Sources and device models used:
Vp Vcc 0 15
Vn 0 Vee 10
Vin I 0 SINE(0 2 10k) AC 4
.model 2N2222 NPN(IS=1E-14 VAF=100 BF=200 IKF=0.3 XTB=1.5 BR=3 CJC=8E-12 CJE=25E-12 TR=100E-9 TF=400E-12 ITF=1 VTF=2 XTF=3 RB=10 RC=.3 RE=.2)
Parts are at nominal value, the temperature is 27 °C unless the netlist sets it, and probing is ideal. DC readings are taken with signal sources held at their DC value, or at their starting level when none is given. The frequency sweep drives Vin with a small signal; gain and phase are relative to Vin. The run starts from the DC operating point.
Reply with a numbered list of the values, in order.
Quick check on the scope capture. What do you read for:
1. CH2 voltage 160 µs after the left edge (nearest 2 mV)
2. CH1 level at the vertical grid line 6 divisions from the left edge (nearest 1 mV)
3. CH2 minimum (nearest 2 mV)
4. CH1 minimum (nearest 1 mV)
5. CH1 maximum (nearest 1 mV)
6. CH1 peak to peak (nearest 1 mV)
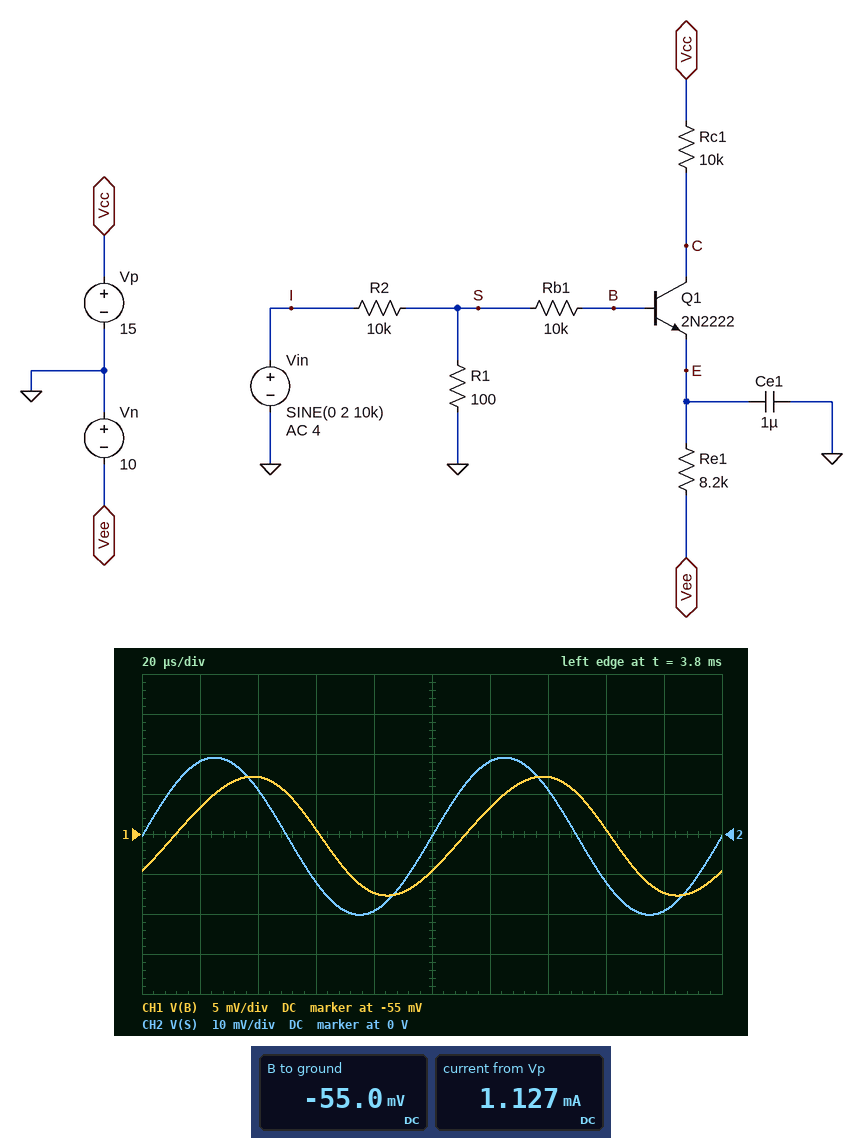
1. -12 mV
2. -52 mV
3. -20 mV
4. -63 mV
5. -48 mV
6. 15 mV
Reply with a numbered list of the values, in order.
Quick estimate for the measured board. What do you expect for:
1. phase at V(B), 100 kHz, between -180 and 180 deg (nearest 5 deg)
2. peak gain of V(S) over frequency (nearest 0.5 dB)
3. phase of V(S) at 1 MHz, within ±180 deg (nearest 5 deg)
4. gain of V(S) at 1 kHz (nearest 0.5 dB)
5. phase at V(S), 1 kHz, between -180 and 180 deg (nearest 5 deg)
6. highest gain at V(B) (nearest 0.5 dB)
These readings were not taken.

1. -75 deg
2. -40.0 dB
3. 0 deg
4. -40.0 dB
5. 0 deg
6. -40.0 dB
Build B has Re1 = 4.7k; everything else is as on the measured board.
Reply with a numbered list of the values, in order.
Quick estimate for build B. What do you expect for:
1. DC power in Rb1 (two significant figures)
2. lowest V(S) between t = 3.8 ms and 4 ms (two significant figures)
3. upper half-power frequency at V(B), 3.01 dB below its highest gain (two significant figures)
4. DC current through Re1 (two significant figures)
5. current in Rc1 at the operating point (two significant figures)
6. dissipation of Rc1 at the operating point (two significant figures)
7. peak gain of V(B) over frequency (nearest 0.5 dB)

1. 100 µW
2. -30 mV
3. 66 Hz
4. 1.8 mA
5. 1.7 mA
6. 28 mW
7. -52.0 dB
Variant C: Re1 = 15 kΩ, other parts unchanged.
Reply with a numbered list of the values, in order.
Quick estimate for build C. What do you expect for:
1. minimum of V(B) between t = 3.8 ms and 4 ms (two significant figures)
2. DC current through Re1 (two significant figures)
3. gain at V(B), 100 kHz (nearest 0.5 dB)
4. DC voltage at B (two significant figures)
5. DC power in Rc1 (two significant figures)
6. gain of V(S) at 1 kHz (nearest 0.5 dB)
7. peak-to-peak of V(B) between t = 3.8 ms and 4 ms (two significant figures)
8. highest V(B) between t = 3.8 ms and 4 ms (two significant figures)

1. -39 mV
2. 620 µA
3. -55.0 dB
4. -29 mV
5. 3.8 mW
6. -40.0 dB
7. 20 mV
8. -19 mV
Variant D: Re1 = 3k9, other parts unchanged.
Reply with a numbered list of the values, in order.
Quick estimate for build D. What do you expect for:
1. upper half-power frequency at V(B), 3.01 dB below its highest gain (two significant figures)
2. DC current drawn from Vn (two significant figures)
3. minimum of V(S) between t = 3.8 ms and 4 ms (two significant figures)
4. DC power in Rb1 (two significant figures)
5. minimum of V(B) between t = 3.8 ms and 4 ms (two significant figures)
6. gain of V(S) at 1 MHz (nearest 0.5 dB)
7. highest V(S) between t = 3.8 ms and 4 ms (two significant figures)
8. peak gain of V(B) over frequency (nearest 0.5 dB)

1. 73 Hz
2. 1.9 mA
3. -37 mV
4. 320 µW
5. -1.8 V
6. -40.0 dB
7. 1.8 mV
8. -53.0 dB
